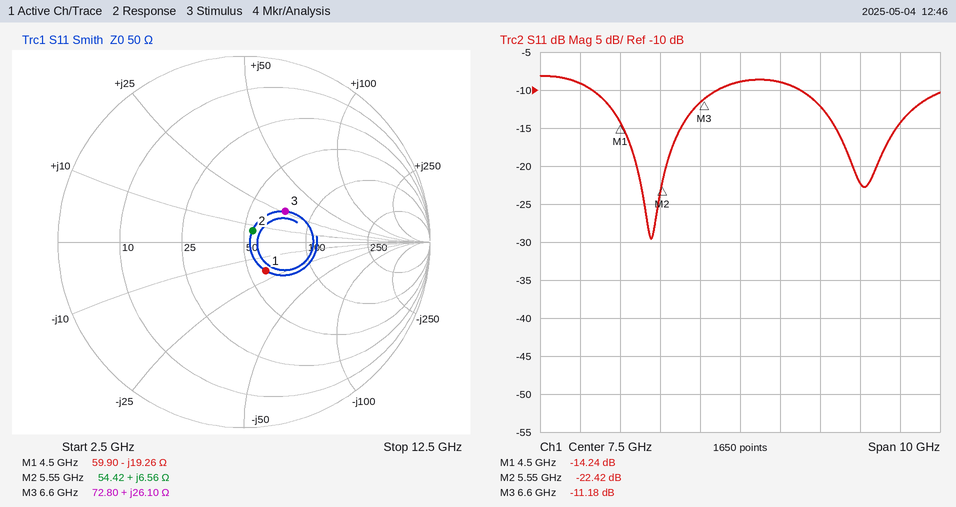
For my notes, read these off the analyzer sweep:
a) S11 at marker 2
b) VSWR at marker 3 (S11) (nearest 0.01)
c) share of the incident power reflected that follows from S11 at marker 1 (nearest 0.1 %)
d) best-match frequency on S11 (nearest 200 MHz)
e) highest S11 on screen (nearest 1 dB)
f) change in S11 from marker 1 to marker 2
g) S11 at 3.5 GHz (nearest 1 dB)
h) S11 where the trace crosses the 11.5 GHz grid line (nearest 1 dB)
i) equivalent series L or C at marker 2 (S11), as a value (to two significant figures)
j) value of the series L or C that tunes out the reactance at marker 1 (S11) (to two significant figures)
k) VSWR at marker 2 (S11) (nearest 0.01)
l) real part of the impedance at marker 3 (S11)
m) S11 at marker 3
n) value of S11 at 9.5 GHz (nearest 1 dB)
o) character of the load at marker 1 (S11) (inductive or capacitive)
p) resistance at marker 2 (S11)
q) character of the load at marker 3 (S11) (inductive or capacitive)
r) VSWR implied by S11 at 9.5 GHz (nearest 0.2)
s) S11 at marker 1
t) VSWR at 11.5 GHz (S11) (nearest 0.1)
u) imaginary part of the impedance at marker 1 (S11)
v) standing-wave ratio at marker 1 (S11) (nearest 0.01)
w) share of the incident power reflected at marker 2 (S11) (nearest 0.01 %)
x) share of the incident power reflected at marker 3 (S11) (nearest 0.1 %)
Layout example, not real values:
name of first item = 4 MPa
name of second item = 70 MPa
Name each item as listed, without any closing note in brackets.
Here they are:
S11 at marker 2 = -22.42 dB
VSWR at marker 3 (S11) = 1.76
share of the incident power reflected that follows from S11 at marker 1 = 3.8 %
best-match frequency on S11 = 5.2 GHz
highest S11 on screen = -8 dB
change in S11 from marker 1 to marker 2 = -8.18 dB
S11 at 3.5 GHz = -9 dB
S11 where the trace crosses the 11.5 GHz grid line = -14 dB
equivalent series L or C at marker 2 (S11), as a value = 190 pH
value of the series L or C that tunes out the reactance at marker 1 (S11) = 680 pH
VSWR at marker 2 (S11) = 1.16
real part of the impedance at marker 3 = 72.80 Ω
S11 at marker 3 = -11.18 dB
value of S11 at 9.5 GHz = -12 dB
character of the load at marker 1 (S11) = capacitive
resistance at marker 2 = 54.42 Ω
character of the load at marker 3 (S11) = inductive
VSWR implied by S11 at 9.5 GHz = 1.6
S11 at marker 1 = -14.24 dB
VSWR at 11.5 GHz (S11) = 1.5
imaginary part of the impedance at marker 1 = -19.26 Ω
standing-wave ratio at marker 1 (S11) = 1.48
share of the incident power reflected at marker 2 (S11) = 0.57 %
share of the incident power reflected at marker 3 (S11) = 7.6 %
